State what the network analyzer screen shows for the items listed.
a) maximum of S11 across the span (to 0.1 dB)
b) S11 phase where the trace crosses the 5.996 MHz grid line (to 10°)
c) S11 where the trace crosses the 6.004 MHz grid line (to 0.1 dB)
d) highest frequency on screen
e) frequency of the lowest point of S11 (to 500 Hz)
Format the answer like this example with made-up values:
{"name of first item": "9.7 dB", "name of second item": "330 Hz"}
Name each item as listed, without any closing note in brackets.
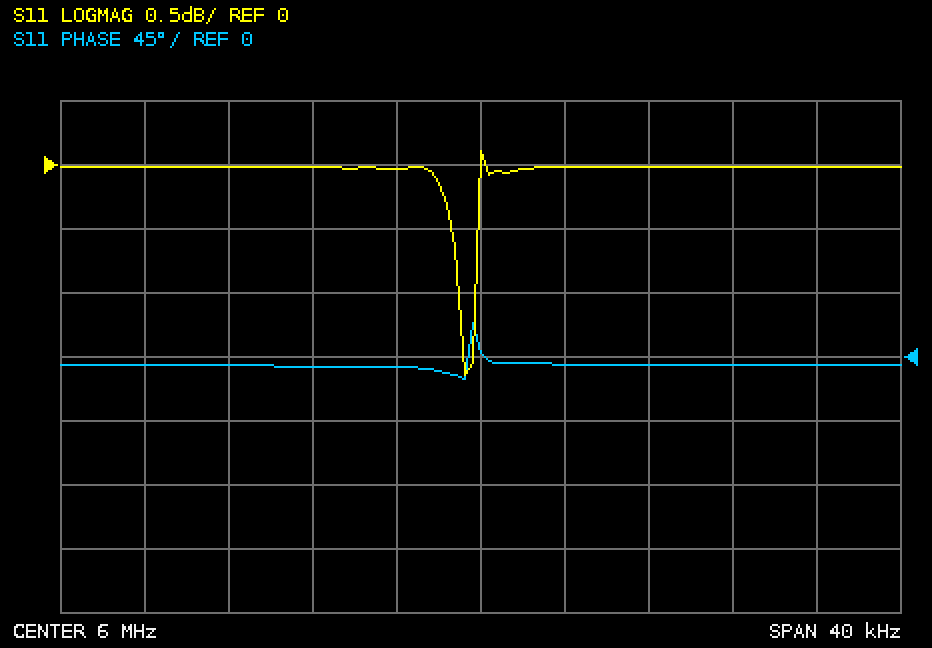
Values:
{"maximum of S11 across the span": "0.1 dB", "S11 phase where the trace crosses the 5.996 MHz grid line": "-10°", "S11 where the trace crosses the 6.004 MHz grid line": "0.0 dB", "highest frequency on screen": "6.02 MHz", "frequency of the lowest point of S11": "5.9990 MHz"}
